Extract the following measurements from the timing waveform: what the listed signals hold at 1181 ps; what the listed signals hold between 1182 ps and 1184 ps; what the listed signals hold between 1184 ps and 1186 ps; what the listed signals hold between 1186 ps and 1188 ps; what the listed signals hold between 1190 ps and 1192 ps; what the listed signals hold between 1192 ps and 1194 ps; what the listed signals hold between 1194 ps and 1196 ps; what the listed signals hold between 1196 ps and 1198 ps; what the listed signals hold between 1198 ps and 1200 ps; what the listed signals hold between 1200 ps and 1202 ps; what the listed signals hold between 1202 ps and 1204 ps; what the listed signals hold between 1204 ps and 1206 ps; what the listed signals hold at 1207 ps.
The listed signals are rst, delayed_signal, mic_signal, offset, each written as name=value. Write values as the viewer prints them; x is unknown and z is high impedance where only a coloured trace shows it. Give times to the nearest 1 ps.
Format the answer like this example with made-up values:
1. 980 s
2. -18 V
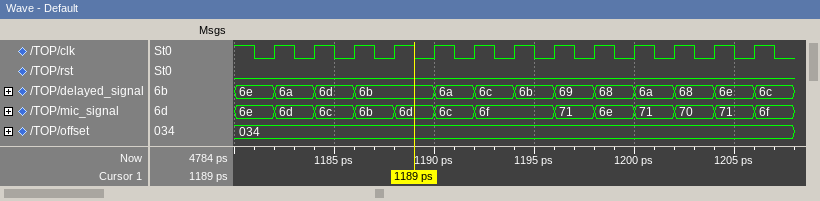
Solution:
1. rst=0, delayed_signal=6e, mic_signal=6e, offset=034
2. rst=0, delayed_signal=6a, mic_signal=6d, offset=034
3. rst=0, delayed_signal=6d, mic_signal=6c, offset=034
4. rst=0, delayed_signal=6b, mic_signal=6b, offset=034
5. rst=0, delayed_signal=6a, mic_signal=6c, offset=034
6. rst=0, delayed_signal=6c, mic_signal=6f, offset=034
7. rst=0, delayed_signal=6b, mic_signal=6f, offset=034
8. rst=0, delayed_signal=69, mic_signal=71, offset=034
9. rst=0, delayed_signal=68, mic_signal=6e, offset=034
10. rst=0, delayed_signal=6a, mic_signal=71, offset=034
11. rst=0, delayed_signal=68, mic_signal=70, offset=034
12. rst=0, delayed_signal=6e, mic_signal=71, offset=034
13. rst=0, delayed_signal=6c, mic_signal=6f, offset=034
